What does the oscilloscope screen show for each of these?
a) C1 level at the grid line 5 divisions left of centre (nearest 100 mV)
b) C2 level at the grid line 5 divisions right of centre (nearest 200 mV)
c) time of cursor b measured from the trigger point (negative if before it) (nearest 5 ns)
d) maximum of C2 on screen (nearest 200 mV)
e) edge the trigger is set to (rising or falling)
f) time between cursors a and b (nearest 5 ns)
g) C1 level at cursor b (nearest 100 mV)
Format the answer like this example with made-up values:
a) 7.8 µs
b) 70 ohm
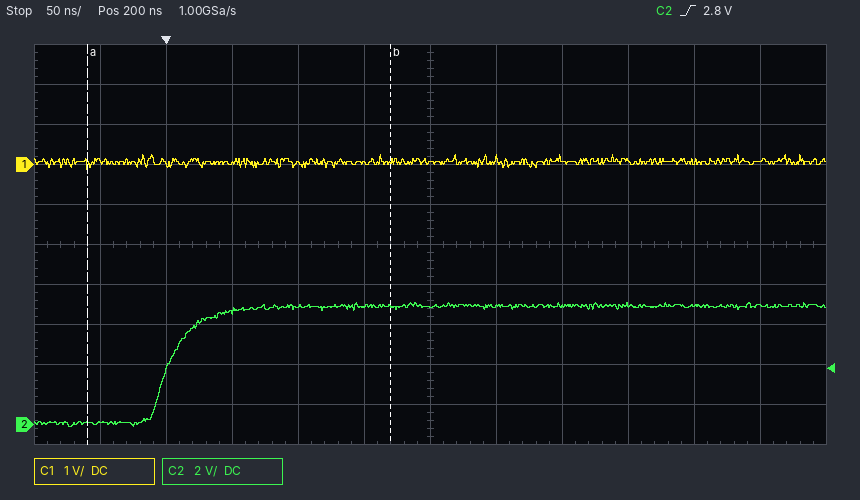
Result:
a) 100 mV
b) 6.0 V
c) +170 ns
d) 6.0 V
e) rising
f) 230 ns
g) 100 mV
